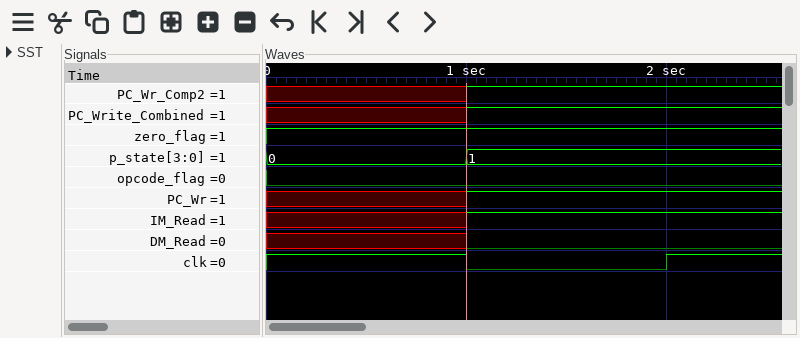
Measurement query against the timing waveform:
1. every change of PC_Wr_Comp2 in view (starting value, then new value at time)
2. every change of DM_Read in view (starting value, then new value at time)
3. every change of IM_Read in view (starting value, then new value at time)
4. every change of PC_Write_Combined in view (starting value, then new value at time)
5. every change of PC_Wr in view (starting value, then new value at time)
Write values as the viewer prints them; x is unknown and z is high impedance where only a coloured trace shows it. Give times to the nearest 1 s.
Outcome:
x, 1 at 1 s
x, 0 at 1 s
x, 1 at 1 s
x, 1 at 1 s
x, 1 at 1 s
